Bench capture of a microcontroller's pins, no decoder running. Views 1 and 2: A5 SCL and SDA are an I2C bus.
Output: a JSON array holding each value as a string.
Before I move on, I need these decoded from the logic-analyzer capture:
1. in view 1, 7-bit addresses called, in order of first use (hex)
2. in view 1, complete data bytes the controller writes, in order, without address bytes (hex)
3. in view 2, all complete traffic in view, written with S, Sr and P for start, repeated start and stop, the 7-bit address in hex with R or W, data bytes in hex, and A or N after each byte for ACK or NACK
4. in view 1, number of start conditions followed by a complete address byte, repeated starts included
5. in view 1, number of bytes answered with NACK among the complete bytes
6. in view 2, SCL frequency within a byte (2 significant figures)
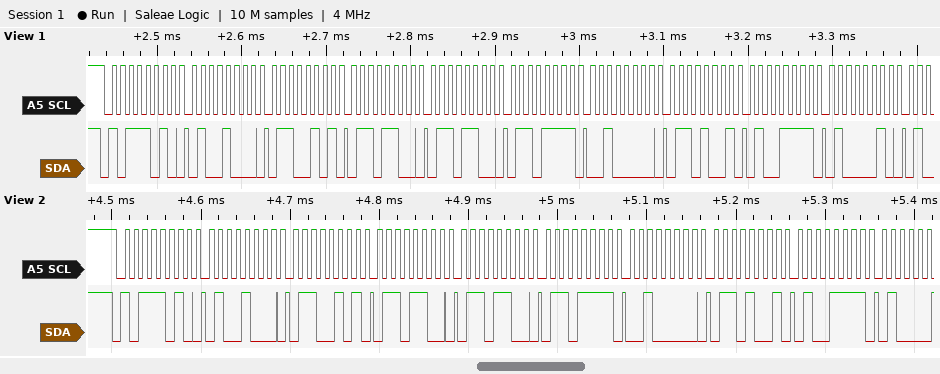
["0x5D", "48 65 6C 6C 6F 20 69 4F 42", "S 5DW A 48 A 65 A 6C A 6C A 6F A 20 A 69 A 4F A", "1", "0", "100 kHz"]
